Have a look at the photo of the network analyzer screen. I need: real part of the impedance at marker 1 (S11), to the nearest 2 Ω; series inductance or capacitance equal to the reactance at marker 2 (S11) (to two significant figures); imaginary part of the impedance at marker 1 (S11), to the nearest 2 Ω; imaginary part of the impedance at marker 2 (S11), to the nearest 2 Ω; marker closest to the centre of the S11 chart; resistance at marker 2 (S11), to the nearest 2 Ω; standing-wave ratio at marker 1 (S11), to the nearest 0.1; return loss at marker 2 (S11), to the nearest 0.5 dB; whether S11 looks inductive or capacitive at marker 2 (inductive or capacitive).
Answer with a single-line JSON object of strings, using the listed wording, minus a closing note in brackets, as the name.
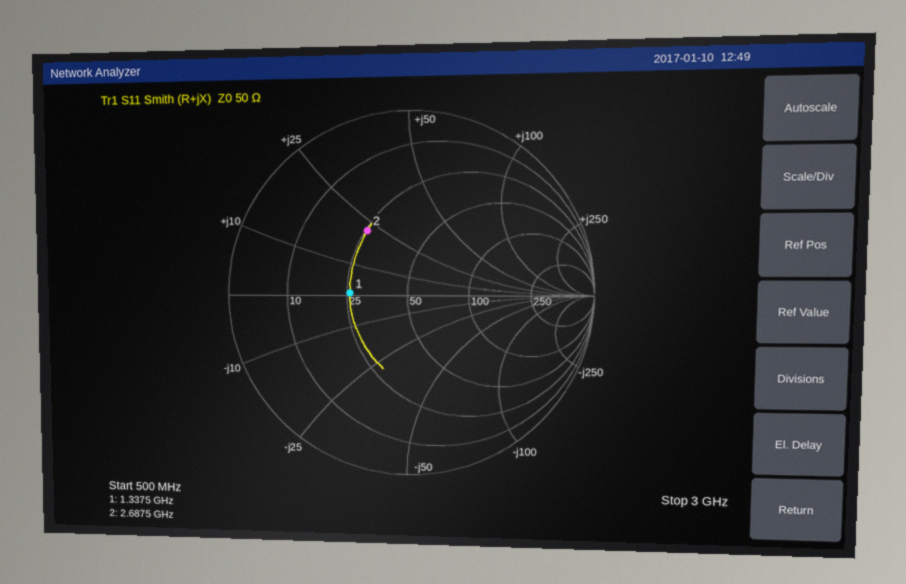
{"real part of the impedance at marker 1 (S11), to the nearest 2 Ω": "26 Ω", "series inductance or capacitance equal to the reactance at marker 2 (S11)": "1.3 nH", "imaginary part of the impedance at marker 1 (S11), to the nearest 2 Ω": "0 Ω", "imaginary part of the impedance at marker 2 (S11), to the nearest 2 Ω": "+22 Ω", "marker closest to the centre of the S11 chart": "marker 1", "resistance at marker 2 (S11), to the nearest 2 Ω": "26 Ω", "standing-wave ratio at marker 1 (S11), to the nearest 0.1": "1.9", "return loss at marker 2 (S11), to the nearest 0.5 dB": "7.5 dB", "whether S11 looks inductive or capacitive at marker 2": "inductive"}
